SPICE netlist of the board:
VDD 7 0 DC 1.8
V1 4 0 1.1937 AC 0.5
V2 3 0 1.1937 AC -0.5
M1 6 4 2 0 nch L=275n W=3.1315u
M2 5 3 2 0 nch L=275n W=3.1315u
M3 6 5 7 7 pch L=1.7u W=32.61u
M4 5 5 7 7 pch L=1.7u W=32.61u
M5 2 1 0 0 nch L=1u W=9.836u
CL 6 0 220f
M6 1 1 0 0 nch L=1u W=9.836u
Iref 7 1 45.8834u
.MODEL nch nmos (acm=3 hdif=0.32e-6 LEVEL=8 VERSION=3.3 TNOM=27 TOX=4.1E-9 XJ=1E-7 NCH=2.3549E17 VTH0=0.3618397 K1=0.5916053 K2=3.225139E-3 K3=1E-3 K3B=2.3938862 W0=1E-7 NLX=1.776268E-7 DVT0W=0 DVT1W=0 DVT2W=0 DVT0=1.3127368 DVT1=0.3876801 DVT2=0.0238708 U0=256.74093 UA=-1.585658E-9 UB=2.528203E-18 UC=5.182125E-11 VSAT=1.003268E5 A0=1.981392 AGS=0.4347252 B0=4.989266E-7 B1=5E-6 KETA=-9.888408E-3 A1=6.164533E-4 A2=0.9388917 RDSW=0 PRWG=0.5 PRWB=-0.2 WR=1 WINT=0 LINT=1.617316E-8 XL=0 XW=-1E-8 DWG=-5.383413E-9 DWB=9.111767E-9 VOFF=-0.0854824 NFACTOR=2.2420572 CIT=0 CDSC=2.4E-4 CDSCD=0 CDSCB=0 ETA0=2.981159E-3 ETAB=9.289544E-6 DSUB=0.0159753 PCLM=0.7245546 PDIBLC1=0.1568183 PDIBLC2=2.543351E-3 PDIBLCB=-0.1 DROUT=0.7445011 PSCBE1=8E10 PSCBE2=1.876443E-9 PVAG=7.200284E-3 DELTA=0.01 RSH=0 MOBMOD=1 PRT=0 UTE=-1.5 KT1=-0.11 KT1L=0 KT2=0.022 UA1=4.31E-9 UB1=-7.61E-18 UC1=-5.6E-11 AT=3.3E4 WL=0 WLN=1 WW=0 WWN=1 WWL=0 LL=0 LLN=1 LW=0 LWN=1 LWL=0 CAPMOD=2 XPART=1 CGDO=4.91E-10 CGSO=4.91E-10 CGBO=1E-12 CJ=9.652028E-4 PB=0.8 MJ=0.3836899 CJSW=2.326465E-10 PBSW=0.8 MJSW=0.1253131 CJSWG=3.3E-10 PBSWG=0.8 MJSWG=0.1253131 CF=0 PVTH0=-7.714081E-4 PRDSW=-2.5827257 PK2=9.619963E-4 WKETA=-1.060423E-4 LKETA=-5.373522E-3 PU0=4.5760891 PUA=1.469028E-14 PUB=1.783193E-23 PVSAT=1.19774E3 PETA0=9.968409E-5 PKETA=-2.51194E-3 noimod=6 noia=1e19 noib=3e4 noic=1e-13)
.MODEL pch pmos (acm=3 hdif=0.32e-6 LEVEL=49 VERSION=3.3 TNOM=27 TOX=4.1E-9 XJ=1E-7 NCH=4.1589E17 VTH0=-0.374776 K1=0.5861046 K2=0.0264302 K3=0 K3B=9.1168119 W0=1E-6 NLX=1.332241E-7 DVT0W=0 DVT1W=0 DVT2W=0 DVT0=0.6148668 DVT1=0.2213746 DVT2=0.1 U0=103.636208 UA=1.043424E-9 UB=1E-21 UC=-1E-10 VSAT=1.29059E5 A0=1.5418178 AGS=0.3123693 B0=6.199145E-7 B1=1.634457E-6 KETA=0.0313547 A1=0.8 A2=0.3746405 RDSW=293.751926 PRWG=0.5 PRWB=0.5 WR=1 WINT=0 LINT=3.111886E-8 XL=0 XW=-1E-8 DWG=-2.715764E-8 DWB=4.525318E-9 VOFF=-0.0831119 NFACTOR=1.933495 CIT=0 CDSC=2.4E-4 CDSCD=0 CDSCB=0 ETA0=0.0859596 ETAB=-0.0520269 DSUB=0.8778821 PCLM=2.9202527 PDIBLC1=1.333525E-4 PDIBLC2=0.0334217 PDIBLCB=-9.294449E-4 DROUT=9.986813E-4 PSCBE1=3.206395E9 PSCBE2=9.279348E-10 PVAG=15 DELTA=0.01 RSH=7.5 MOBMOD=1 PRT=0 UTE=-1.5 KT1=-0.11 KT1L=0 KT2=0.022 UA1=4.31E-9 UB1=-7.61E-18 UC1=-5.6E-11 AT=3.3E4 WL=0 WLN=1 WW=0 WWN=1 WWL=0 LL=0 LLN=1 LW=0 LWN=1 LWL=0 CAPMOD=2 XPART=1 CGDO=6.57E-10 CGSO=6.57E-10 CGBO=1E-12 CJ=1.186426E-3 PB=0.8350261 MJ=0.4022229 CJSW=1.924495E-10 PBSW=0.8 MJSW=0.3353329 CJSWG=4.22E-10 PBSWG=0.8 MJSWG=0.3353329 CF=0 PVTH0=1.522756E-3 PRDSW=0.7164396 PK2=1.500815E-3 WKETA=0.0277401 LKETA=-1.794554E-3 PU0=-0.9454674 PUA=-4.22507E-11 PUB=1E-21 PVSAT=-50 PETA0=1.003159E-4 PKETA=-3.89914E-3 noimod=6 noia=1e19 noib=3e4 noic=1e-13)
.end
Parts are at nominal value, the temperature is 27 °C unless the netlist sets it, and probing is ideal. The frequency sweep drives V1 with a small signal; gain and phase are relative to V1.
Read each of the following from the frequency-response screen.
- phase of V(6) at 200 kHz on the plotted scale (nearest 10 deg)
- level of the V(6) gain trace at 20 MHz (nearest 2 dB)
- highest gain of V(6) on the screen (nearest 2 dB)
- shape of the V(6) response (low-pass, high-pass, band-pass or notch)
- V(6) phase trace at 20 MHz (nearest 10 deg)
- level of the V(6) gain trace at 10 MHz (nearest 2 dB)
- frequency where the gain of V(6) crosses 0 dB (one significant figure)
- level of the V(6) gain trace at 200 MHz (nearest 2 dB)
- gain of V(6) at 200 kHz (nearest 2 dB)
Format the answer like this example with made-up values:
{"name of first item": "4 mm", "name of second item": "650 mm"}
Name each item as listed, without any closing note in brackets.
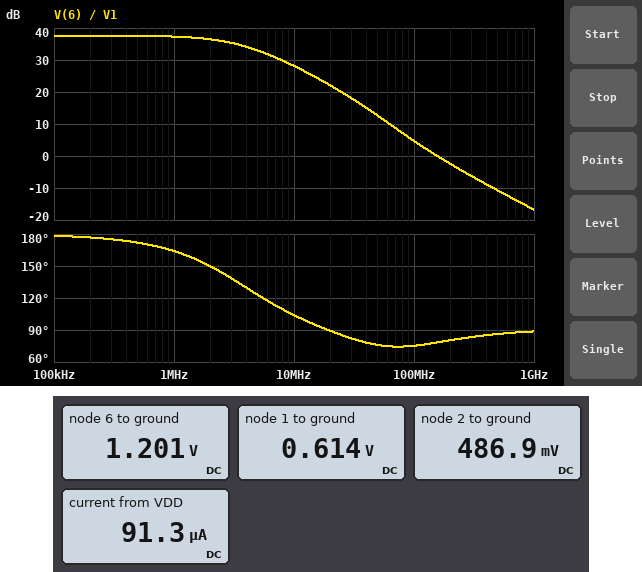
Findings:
{"phase of V(6) at 200 kHz on the plotted scale": "180 deg", "level of the V(6) gain trace at 20 MHz": "22 dB", "highest gain of V(6) on the screen": "38 dB", "shape of the V(6) response": "low-pass", "V(6) phase trace at 20 MHz": "90 deg", "level of the V(6) gain trace at 10 MHz": "28 dB", "frequency where the gain of V(6) crosses 0 dB": "200 MHz", "level of the V(6) gain trace at 200 MHz": "-2 dB", "gain of V(6) at 200 kHz": "38 dB"}
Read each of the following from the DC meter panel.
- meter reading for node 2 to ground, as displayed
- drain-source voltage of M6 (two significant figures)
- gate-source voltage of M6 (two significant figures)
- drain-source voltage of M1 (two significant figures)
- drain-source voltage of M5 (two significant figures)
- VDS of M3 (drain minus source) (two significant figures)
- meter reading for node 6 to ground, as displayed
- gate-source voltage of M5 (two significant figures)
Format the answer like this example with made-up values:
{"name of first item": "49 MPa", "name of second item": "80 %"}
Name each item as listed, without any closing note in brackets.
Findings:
{"meter reading for node 2 to ground, as displayed": "486.9 mV", "drain-source voltage of M6": "610 mV", "gate-source voltage of M6": "610 mV", "drain-source voltage of M1": "710 mV", "drain-source voltage of M5": "490 mV", "VDS of M3 (drain minus source)": "-600 mV", "meter reading for node 6 to ground, as displayed": "1.201 V", "gate-source voltage of M5": "610 mV"}
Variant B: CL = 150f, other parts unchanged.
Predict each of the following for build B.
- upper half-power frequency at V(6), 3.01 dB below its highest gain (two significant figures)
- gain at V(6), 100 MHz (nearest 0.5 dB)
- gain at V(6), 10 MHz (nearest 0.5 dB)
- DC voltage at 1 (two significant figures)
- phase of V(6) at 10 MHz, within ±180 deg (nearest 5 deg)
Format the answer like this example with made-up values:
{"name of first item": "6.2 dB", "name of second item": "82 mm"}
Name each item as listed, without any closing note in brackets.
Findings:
{"upper half-power frequency at V(6), 3.01 dB below its highest gain": "4.7 MHz", "gain at V(6), 100 MHz": "7.0 dB", "gain at V(6), 10 MHz": "30.0 dB", "DC voltage at 1": "610 mV", "phase of V(6) at 10 MHz, within ±180 deg": "110 deg"}
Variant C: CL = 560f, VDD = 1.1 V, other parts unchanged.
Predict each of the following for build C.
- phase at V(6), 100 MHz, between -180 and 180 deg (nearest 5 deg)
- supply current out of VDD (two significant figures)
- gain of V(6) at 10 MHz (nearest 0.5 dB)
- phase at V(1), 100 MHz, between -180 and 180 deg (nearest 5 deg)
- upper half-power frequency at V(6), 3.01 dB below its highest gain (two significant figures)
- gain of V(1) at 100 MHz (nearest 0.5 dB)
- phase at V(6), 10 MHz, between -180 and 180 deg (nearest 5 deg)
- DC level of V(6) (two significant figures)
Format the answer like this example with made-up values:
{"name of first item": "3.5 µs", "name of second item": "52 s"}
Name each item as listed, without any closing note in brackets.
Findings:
{"phase at V(6), 100 MHz, between -180 and 180 deg": "105 deg", "supply current out of VDD": "91 µA", "gain of V(6) at 10 MHz": "0 dB", "phase at V(1), 100 MHz, between -180 and 180 deg": "110 deg", "upper half-power frequency at V(6), 3.01 dB below its highest gain": "46 MHz", "gain of V(1) at 100 MHz": "-61.5 dB", "phase at V(6), 10 MHz, between -180 and 180 deg": "165 deg", "DC level of V(6)": "500 mV"}
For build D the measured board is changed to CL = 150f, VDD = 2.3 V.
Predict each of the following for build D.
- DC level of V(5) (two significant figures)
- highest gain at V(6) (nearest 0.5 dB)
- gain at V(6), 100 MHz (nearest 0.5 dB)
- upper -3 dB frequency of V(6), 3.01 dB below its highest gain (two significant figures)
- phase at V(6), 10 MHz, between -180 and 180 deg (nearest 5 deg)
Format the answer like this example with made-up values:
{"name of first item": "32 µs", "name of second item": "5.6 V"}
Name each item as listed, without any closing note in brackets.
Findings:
{"DC level of V(5)": "1.7 V", "highest gain at V(6)": "38.0 dB", "gain at V(6), 100 MHz": "7.0 dB", "upper -3 dB frequency of V(6), 3.01 dB below its highest gain": "4.5 MHz", "phase at V(6), 10 MHz, between -180 and 180 deg": "110 deg"}
